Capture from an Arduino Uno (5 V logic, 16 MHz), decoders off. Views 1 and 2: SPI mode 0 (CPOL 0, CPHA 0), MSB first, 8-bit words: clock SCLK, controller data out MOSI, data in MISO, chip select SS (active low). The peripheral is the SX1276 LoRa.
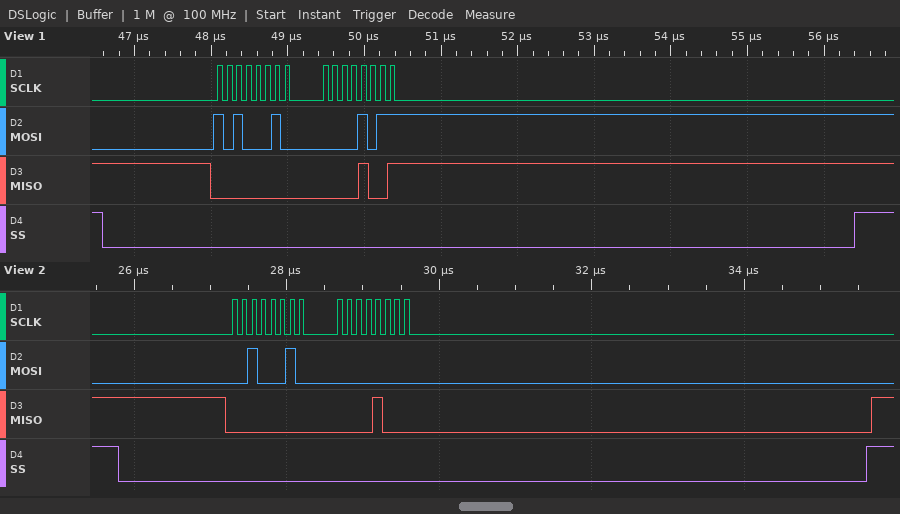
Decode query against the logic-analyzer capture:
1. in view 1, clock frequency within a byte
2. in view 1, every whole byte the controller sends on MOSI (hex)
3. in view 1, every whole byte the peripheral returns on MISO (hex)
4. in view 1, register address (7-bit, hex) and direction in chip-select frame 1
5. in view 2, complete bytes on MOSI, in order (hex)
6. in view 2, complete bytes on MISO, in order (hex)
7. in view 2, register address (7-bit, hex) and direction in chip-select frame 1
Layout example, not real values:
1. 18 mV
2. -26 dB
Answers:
1. 8 MHz
2. A2 0B
3. 00 09
4. 0x22 write
5. 22 00
6. 00 08
7. 0x22 read
